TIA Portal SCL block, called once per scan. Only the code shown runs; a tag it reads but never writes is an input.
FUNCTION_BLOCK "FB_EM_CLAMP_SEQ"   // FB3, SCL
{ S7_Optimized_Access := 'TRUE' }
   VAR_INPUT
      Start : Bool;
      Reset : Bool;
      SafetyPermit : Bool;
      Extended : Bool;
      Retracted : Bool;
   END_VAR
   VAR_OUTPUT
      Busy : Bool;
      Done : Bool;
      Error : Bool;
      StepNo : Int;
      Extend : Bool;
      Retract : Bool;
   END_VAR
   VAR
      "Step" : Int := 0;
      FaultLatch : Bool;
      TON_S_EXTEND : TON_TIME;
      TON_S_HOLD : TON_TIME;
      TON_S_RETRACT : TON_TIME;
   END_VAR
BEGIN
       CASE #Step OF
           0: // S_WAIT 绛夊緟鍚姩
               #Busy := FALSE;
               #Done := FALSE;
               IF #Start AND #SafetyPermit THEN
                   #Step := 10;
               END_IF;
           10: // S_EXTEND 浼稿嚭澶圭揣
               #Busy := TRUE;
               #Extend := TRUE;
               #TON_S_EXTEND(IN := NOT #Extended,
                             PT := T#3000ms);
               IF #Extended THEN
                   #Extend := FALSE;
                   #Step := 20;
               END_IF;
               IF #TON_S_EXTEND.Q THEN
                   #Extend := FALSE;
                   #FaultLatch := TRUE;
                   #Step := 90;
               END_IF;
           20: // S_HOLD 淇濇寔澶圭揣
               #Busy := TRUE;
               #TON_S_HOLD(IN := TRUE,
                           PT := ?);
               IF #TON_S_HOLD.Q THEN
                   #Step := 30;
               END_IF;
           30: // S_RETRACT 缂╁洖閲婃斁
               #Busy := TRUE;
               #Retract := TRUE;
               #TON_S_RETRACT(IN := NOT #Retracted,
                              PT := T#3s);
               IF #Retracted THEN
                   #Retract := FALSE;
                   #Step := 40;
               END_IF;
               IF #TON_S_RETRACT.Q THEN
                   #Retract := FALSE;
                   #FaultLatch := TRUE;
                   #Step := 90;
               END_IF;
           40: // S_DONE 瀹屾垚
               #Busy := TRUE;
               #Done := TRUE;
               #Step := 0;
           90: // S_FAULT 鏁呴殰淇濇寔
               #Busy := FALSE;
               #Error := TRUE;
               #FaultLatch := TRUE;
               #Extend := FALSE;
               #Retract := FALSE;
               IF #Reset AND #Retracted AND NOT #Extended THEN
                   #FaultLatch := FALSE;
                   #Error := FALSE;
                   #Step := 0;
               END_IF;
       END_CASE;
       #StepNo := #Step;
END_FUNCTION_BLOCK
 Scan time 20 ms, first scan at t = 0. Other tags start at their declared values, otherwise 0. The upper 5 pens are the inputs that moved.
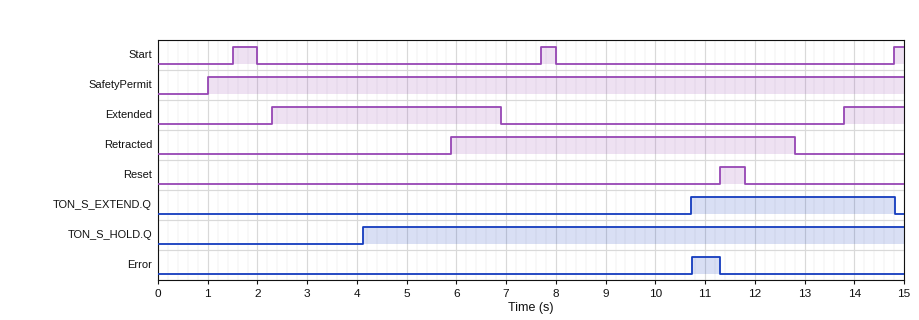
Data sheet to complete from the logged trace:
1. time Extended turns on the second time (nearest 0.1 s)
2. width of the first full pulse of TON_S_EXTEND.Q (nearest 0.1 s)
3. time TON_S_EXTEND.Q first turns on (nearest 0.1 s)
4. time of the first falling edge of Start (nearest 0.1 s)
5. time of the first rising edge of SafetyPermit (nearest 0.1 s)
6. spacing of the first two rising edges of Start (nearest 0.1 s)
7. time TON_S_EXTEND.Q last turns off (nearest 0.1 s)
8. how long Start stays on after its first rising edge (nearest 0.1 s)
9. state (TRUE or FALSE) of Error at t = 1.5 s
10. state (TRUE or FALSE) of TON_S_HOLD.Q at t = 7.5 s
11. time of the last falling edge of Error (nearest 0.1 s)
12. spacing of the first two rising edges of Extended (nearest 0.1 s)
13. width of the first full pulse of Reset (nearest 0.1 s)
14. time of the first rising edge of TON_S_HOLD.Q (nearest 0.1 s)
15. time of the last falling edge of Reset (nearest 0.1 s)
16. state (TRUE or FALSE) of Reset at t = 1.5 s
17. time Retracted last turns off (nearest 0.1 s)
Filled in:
13.8 s
4.1 s
10.7 s
2.0 s
1.0 s
6.2 s
14.8 s
0.5 s
FALSE
TRUE
11.3 s
11.5 s
0.5 s
4.1 s
11.8 s
FALSE
12.8 s
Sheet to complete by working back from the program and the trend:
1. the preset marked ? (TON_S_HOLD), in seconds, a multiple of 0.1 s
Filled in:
1.8 s
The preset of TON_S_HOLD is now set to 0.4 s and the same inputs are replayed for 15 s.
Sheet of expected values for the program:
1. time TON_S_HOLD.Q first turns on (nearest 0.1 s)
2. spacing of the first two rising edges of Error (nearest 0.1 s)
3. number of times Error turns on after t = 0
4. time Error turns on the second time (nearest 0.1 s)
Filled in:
2.7 s
9.1 s
2
14.9 s
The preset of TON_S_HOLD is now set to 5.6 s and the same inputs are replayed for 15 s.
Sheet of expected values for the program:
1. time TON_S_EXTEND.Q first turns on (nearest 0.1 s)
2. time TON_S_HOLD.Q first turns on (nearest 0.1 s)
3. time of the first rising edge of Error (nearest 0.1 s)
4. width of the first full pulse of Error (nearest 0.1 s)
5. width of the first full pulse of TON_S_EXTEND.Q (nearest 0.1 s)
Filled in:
11.0 s
7.9 s
11.0 s
0.3 s
3.8 s
